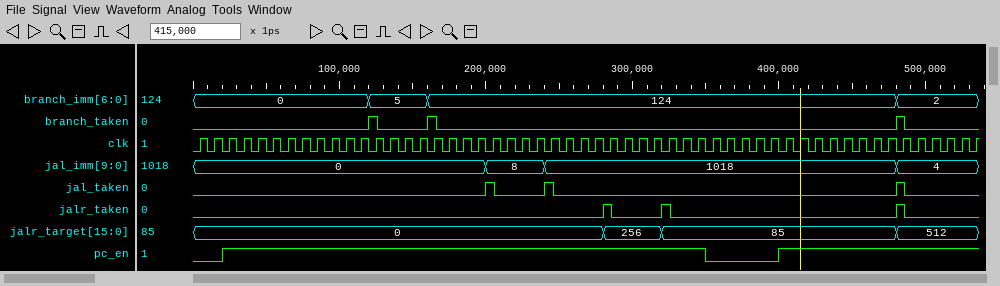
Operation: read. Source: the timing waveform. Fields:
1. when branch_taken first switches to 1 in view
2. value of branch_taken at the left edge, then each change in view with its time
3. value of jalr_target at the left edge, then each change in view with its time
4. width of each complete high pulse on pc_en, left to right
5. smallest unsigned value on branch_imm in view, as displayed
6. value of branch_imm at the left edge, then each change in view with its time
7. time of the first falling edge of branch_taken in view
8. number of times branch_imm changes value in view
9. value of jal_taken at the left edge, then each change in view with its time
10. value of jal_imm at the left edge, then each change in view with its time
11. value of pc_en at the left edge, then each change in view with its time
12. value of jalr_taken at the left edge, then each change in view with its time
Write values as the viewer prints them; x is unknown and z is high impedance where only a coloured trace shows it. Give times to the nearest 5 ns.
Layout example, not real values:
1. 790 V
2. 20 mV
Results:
1. 120 ns
2. 0, 1 at 120 ns, 0 at 125 ns, 1 at 160 ns, 0 at 165 ns, 1 at 480 ns, 0 at 485 ns
3. 0, 256 at 280 ns, 85 at 320 ns, 512 at 480 ns
4. 330 ns
5. 0
6. 0, 5 at 120 ns, 124 at 160 ns, 2 at 480 ns
7. 125 ns
8. 3
9. 0, 1 at 200 ns, 0 at 205 ns, 1 at 240 ns, 0 at 245 ns, 1 at 480 ns, 0 at 485 ns
10. 0, 8 at 200 ns, 1018 at 240 ns, 4 at 480 ns
11. 0, 1 at 20 ns, 0 at 350 ns, 1 at 400 ns
12. 0, 1 at 280 ns, 0 at 285 ns, 1 at 320 ns, 0 at 325 ns, 1 at 480 ns, 0 at 485 ns
